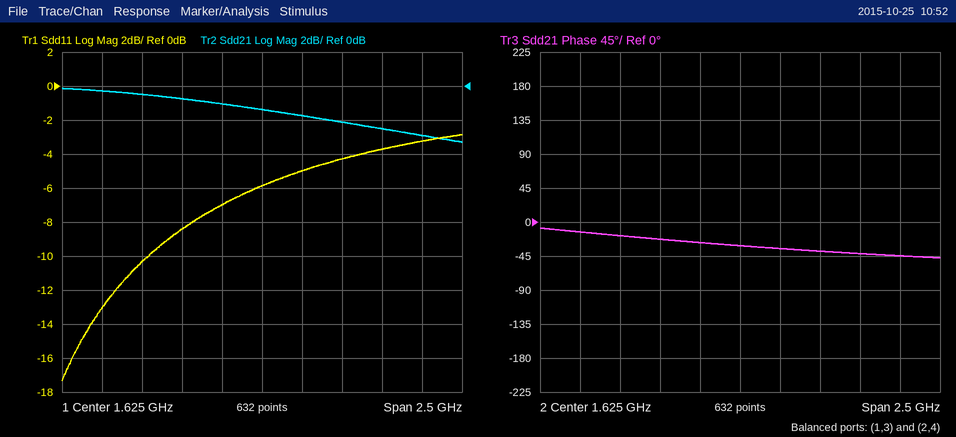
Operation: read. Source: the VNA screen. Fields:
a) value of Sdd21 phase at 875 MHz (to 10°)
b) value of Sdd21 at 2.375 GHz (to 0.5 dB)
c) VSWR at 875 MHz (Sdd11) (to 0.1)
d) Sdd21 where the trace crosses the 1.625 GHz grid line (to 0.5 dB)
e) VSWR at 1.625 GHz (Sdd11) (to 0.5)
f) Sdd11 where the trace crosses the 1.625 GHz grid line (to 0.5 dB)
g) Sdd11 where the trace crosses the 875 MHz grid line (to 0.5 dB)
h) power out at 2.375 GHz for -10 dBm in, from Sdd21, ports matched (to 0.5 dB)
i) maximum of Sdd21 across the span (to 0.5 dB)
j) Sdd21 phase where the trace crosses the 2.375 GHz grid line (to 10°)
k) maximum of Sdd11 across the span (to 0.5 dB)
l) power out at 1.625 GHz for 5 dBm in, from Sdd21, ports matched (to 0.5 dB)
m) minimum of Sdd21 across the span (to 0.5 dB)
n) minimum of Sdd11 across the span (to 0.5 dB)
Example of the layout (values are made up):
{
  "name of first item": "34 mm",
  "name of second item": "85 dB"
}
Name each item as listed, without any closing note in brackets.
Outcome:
{
  "value of Sdd21 phase at 875 MHz": "-20°",
  "value of Sdd21 at 2.375 GHz": "-2.5 dB",
  "VSWR at 875 MHz (Sdd11)": "1.9",
  "Sdd21 where the trace crosses the 1.625 GHz grid line": "-1.5 dB",
  "VSWR at 1.625 GHz (Sdd11)": "3.0",
  "Sdd11 where the trace crosses the 1.625 GHz grid line": "-6.0 dB",
  "Sdd11 where the trace crosses the 875 MHz grid line": "-10.5 dB",
  "power out at 2.375 GHz for -10 dBm in, from Sdd21, ports matched": "-12.5 dBm",
  "maximum of Sdd21 across the span": "0.0 dB",
  "Sdd21 phase where the trace crosses the 2.375 GHz grid line": "-40°",
  "maximum of Sdd11 across the span": "-3.0 dB",
  "power out at 1.625 GHz for 5 dBm in, from Sdd21, ports matched": "3.5 dBm",
  "minimum of Sdd21 across the span": "-3.5 dB",
  "minimum of Sdd11 across the span": "-17.5 dB"
}
